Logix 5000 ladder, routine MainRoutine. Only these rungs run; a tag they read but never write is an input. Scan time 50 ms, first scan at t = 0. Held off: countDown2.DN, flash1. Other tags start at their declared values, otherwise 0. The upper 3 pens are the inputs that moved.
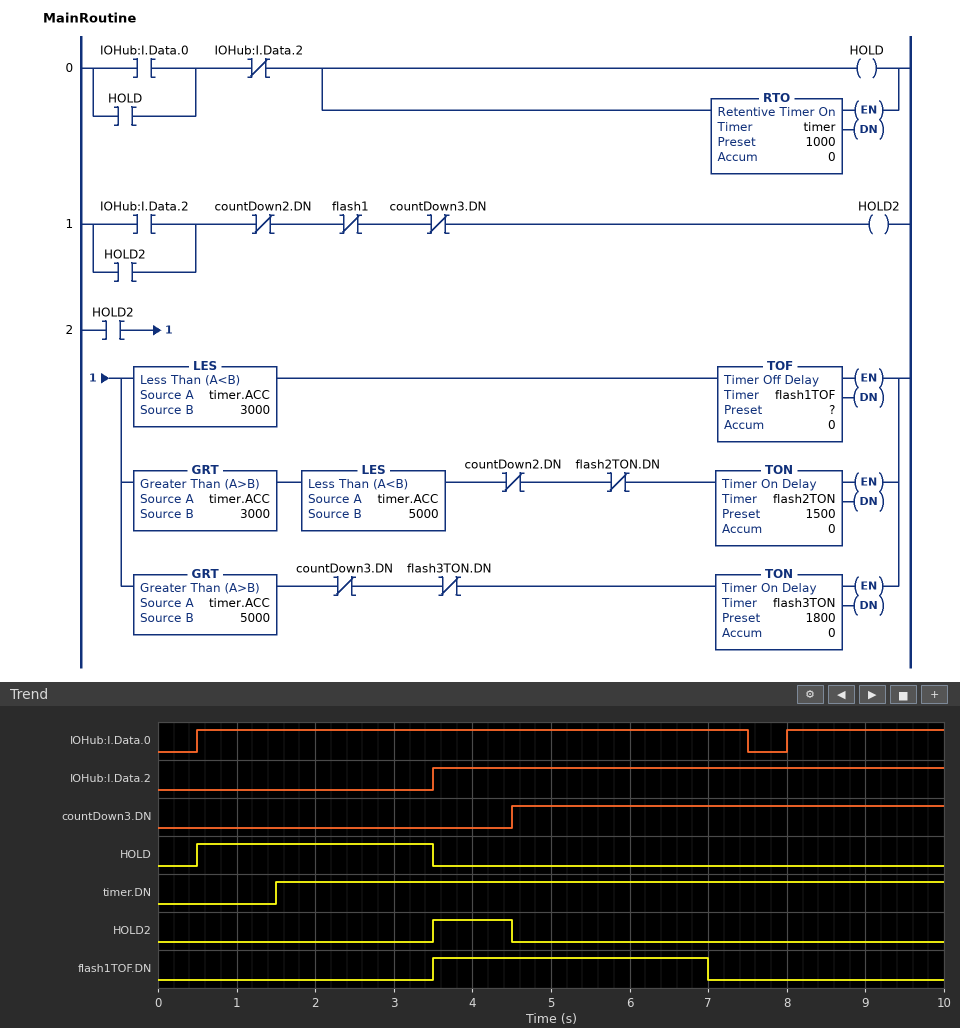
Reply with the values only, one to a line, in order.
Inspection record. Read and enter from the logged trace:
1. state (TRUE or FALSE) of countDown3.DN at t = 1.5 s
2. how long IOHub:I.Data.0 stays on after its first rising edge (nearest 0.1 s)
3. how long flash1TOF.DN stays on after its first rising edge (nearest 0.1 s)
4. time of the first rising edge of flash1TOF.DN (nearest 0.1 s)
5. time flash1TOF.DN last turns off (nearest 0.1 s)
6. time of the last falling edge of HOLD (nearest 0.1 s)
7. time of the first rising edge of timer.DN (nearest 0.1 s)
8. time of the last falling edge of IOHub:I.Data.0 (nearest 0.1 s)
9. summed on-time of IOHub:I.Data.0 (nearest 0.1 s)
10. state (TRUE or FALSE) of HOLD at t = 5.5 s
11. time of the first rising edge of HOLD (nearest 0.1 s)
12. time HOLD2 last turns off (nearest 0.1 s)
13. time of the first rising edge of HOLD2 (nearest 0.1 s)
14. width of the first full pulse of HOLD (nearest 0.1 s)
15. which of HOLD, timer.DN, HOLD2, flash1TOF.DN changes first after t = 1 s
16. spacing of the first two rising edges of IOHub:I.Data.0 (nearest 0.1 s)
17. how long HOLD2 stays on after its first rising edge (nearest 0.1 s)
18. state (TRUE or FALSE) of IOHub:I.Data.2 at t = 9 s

FALSE
7.0 s
3.5 s
3.5 s
7.0 s
3.5 s
1.5 s
7.5 s
9.0 s
FALSE
0.5 s
4.5 s
3.5 s
3.0 s
timer.DN
7.5 s
1.0 s
TRUE
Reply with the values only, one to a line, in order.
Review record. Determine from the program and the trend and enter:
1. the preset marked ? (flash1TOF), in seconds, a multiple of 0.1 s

2.5 s
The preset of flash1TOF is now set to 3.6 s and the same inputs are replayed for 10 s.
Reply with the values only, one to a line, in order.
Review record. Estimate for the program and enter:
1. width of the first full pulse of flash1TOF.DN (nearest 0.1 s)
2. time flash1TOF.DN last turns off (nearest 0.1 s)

4.6 s
8.1 s
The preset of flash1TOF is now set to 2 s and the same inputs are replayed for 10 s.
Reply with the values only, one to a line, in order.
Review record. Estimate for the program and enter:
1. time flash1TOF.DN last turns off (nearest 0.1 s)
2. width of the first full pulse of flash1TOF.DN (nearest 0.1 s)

6.5 s
3.0 s
